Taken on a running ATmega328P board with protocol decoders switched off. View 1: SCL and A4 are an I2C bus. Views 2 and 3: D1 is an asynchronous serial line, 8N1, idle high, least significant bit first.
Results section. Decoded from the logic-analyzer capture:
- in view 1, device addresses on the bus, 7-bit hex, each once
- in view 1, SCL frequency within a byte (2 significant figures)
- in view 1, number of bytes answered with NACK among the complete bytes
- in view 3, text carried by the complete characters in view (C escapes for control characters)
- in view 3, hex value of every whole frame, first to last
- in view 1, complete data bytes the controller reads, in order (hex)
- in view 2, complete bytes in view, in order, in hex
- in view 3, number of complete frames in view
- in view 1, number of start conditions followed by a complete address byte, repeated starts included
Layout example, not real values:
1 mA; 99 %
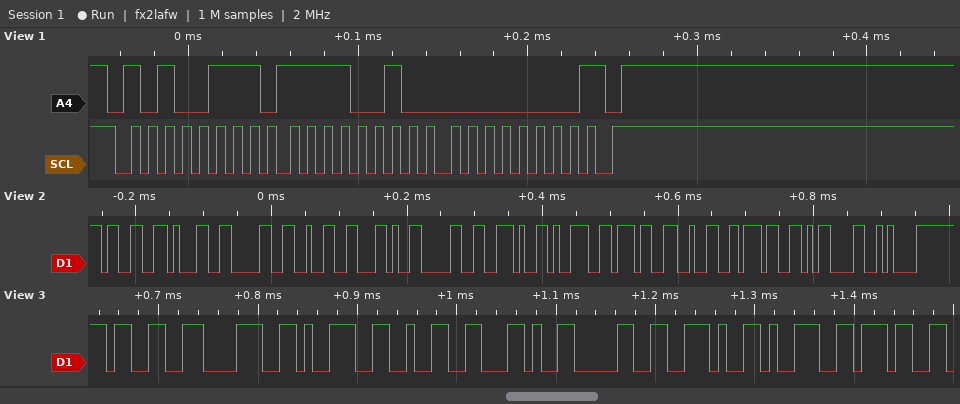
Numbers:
0x53; 100 kHz; 1; "3892,0.97"; 33 38 39 32 2C 30 2E 39 37; F2 00; 33 31 30 32 2C 30 2E 39 37 32 37 0D 0A; 9; 1
